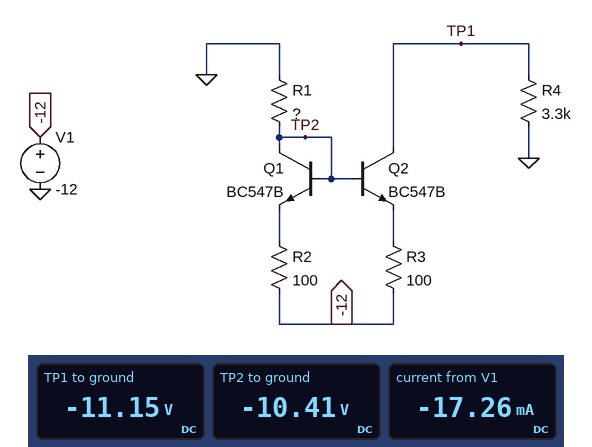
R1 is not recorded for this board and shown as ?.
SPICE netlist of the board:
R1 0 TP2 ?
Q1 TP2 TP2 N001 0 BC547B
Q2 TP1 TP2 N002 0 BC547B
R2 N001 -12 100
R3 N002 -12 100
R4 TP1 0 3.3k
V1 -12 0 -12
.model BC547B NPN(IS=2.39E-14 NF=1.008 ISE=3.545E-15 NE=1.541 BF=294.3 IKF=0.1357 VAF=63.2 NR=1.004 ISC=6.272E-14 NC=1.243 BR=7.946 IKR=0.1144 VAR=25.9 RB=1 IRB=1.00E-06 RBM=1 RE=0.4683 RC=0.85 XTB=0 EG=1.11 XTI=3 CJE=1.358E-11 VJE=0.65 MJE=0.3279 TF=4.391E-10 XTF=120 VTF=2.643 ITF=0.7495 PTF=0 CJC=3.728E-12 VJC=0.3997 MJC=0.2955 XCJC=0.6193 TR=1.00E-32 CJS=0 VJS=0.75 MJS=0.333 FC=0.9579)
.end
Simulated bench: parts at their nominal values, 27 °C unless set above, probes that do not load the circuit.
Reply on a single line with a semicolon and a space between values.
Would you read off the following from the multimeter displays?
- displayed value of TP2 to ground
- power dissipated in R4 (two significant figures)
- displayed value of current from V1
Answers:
-10.41 V; 38 mW; -17.26 mA
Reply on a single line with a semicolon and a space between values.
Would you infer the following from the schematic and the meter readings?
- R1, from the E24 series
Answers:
750 Ω
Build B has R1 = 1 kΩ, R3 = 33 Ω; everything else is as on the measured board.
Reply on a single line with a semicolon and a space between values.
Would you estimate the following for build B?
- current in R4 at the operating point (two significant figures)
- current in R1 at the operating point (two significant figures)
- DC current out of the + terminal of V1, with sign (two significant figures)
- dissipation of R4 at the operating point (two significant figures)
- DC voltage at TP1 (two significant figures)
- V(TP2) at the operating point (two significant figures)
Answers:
3.5 mA; 11 mA; -14 mA; 41 mW; -12 V; -11 V
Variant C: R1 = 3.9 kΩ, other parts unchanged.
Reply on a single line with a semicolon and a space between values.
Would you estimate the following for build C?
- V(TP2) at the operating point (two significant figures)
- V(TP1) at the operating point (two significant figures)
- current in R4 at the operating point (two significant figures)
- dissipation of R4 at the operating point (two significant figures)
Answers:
-11 V; -9.3 V; 2.8 mA; 26 mW
